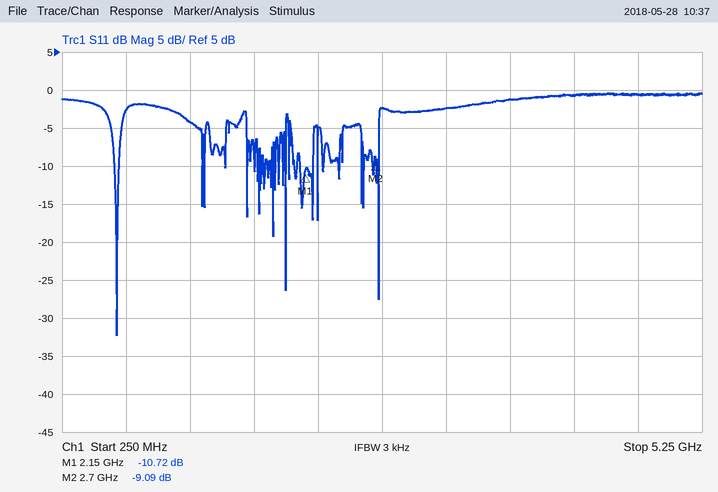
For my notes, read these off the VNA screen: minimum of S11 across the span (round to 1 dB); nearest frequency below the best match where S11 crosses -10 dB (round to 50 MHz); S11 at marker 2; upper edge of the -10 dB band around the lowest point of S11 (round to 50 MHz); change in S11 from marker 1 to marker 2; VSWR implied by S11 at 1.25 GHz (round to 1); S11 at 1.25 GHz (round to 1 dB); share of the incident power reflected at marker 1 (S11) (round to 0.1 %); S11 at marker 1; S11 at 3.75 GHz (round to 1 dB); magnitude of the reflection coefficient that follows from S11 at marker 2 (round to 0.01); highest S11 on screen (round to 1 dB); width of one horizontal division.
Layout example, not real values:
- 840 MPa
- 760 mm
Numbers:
- -32 dB
- 650 MHz
- -9.09 dB
- 700 MHz
- 1.63 dB
- 4
- -4 dB
- 8.5 %
- -10.72 dB
- -1 dB
- 0.35
- 0 dB
- 500 MHz
